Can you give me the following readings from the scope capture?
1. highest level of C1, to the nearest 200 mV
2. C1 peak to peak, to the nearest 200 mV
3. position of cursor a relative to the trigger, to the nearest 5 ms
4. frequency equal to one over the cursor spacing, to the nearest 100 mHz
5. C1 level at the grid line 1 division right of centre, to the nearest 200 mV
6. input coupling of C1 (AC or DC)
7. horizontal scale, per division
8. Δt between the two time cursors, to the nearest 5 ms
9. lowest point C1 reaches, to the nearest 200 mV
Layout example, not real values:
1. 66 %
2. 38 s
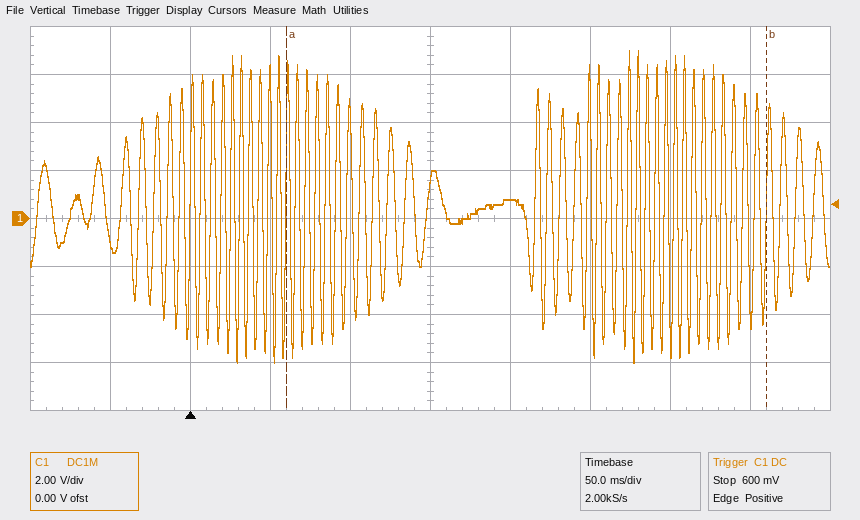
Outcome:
1. 7.0 V
2. 13.0 V
3. +60 ms
4. 3.3 Hz
5. 800 mV
6. DC
7. 50 ms
8. 300 ms
9. -6.0 V
